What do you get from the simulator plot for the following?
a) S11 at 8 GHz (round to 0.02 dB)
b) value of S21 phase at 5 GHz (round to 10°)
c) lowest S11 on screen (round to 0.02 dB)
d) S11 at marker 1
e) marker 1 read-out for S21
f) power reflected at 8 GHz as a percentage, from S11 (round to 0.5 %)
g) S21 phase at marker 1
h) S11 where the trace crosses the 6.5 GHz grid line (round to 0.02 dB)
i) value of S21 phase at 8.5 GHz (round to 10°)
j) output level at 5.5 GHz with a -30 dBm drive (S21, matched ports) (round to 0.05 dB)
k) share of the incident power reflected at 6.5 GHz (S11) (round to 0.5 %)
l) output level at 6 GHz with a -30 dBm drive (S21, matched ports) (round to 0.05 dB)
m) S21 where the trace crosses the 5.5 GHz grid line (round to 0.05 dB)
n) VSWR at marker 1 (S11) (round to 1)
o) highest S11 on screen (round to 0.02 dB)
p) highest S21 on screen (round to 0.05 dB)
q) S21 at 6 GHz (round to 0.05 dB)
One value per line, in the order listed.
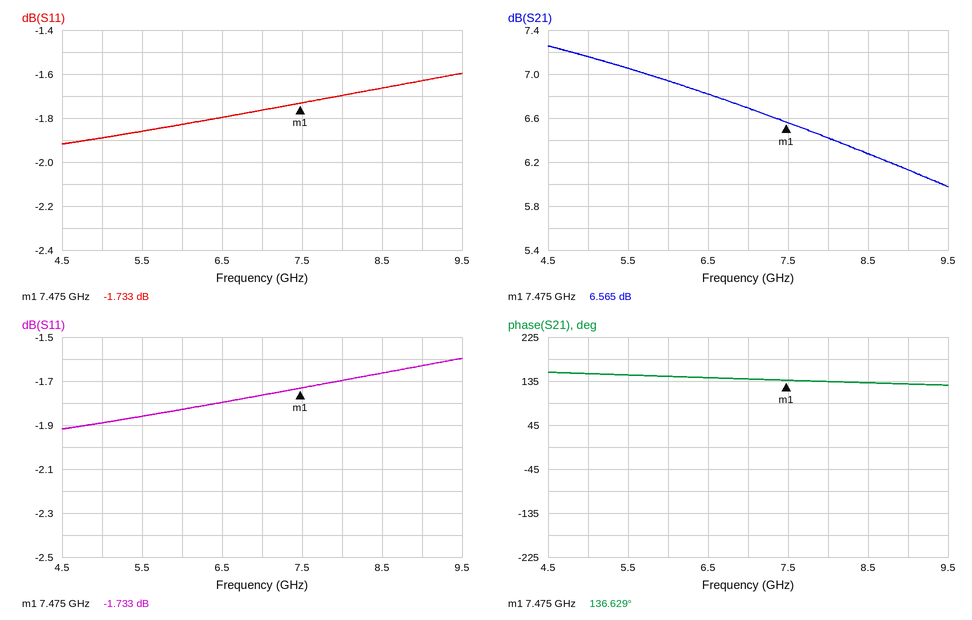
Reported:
-1.70 dB
150°
-1.92 dB
-1.733 dB
6.565 dB
67.5 %
136.629°
-1.80 dB
130°
-22.95 dBm
66.0 %
-23.05 dBm
7.05 dB
10
-1.60 dB
7.25 dB
6.95 dB
